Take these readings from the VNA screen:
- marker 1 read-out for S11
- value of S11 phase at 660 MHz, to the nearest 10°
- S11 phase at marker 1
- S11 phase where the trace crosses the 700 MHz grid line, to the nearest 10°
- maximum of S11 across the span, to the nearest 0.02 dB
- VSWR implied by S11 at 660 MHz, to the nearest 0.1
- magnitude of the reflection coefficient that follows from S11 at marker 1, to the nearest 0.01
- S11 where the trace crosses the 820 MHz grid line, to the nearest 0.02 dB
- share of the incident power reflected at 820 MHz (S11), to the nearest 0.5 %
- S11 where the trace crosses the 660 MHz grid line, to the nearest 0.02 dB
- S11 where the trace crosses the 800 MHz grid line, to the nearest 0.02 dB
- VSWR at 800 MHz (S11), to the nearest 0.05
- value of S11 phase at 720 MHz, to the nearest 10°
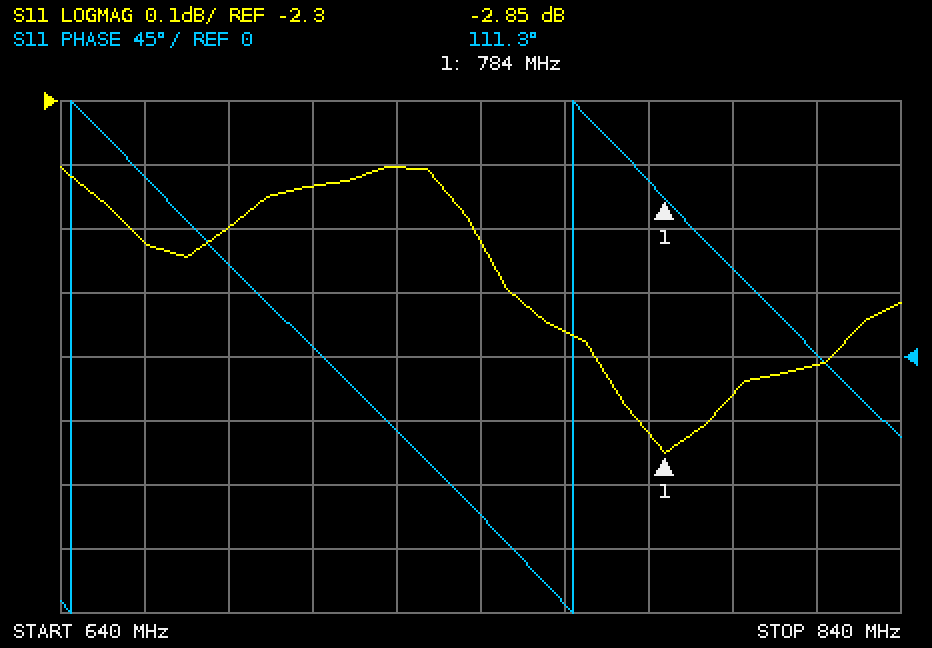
-2.85 dB
130°
111.3°
10°
-2.40 dB
6.9
0.72
-2.72 dB
53.5 %
-2.52 dB
-2.76 dB
6.35
-50°
